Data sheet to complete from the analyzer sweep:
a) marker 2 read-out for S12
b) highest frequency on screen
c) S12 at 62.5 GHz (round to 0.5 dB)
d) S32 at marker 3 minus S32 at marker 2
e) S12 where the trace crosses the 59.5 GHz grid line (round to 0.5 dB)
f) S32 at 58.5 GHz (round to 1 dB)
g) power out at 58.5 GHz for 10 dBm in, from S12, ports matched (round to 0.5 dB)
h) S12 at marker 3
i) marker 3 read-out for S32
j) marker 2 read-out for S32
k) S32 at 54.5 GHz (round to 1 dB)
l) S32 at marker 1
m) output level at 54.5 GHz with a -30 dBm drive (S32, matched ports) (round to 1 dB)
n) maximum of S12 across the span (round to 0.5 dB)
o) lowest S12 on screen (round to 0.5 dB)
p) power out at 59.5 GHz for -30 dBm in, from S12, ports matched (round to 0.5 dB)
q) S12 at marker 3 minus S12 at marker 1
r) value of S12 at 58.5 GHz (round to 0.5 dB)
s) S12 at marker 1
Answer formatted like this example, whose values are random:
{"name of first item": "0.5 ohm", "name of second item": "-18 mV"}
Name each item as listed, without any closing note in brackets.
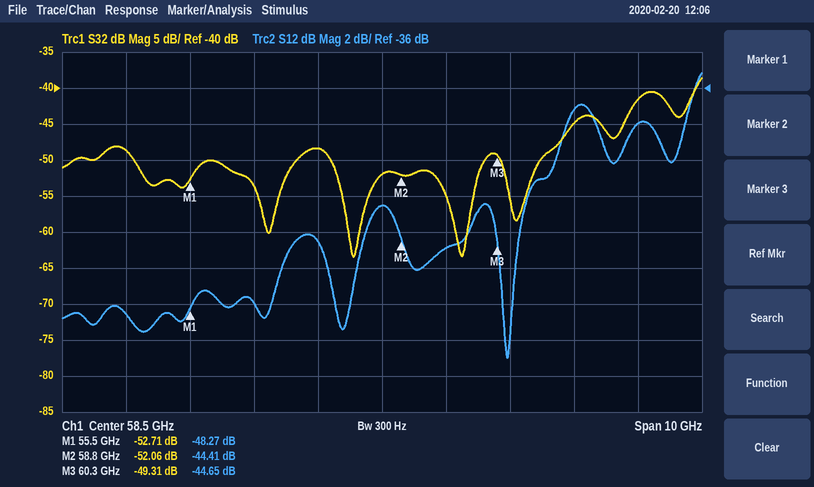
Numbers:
{"marker 2 read-out for S12": "-44.41 dB", "highest frequency on screen": "63.5 GHz", "S12 at 62.5 GHz": "-38.0 dB", "S32 at marker 3 minus S32 at marker 2": "2.75 dB", "S12 where the trace crosses the 59.5 GHz grid line": "-45.0 dB", "S32 at 58.5 GHz": "-52 dB", "power out at 58.5 GHz for 10 dBm in, from S12, ports matched": "-32.5 dBm", "S12 at marker 3": "-44.65 dB", "marker 3 read-out for S32": "-49.31 dB", "marker 2 read-out for S32": "-52.06 dB", "S32 at 54.5 GHz": "-49 dB", "S32 at marker 1": "-52.71 dB", "output level at 54.5 GHz with a -30 dBm drive (S32, matched ports)": "-79 dBm", "maximum of S12 across the span": "-35.0 dB", "lowest S12 on screen": "-51.0 dB", "power out at 59.5 GHz for -30 dBm in, from S12, ports matched": "-75.0 dBm", "S12 at marker 3 minus S12 at marker 1": "3.62 dB", "value of S12 at 58.5 GHz": "-42.5 dB", "S12 at marker 1": "-48.27 dB"}
